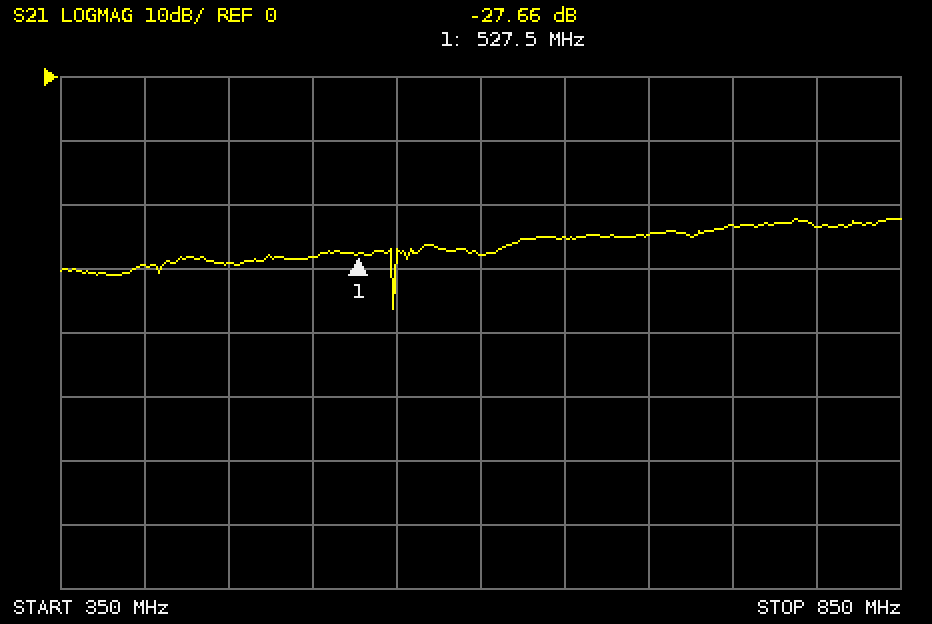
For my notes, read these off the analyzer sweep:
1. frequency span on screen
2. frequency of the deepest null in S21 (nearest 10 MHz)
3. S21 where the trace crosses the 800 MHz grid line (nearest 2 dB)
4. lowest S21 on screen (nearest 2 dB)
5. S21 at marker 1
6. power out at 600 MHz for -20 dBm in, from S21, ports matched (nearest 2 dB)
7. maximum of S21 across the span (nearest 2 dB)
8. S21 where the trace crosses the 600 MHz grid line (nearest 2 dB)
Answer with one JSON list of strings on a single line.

["500 MHz", "550 MHz", "-24 dB", "-36 dB", "-27.66 dB", "-48 dBm", "-22 dB", "-28 dB"]
